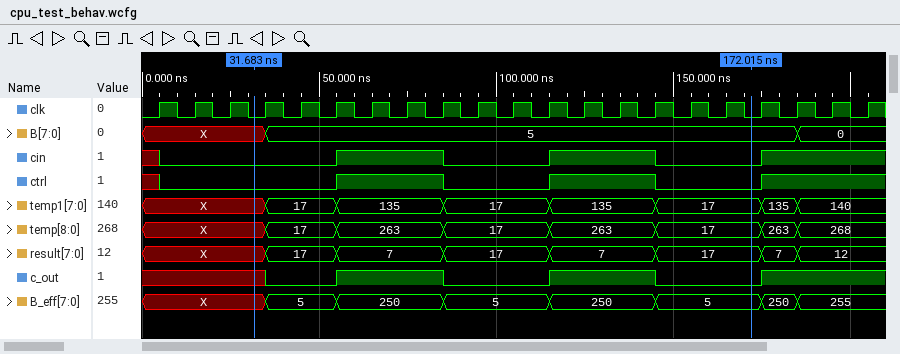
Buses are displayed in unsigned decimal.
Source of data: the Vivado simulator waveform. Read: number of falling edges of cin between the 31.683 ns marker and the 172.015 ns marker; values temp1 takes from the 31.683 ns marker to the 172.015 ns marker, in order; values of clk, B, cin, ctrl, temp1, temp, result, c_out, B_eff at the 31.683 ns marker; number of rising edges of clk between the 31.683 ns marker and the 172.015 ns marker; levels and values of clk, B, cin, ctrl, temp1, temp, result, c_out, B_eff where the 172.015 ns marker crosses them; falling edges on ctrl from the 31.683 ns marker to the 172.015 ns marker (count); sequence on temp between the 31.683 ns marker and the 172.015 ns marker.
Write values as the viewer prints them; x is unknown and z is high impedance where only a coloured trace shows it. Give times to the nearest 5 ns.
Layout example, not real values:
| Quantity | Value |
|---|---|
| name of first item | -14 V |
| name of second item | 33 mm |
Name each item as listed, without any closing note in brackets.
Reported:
| Quantity | Value |
|---|---|
| number of falling edges of cin between the 31.683 ns marker and the 172.015 ns marker | 2 |
| values temp1 takes from the 31.683 ns marker to the 172.015 ns marker, in order | X, 17, 135, 17, 135, 17 |
| values of clk, B, cin, ctrl, temp1, temp, result, c_out, B_eff at the 31.683 ns marker | clk=0, B=X, cin=0, ctrl=0, temp1=X, temp=X, result=X, c_out=x, B_eff=X |
| number of rising edges of clk between the 31.683 ns marker and the 172.015 ns marker | 14 |
| levels and values of clk, B, cin, ctrl, temp1, temp, result, c_out, B_eff where the 172.015 ns marker crosses them | clk=0, B=5, cin=0, ctrl=0, temp1=17, temp=17, result=17, c_out=0, B_eff=5 |
| falling edges on ctrl from the 31.683 ns marker to the 172.015 ns marker | 2 |
| sequence on temp between the 31.683 ns marker and the 172.015 ns marker | X, 17, 263, 17, 263, 17 |
